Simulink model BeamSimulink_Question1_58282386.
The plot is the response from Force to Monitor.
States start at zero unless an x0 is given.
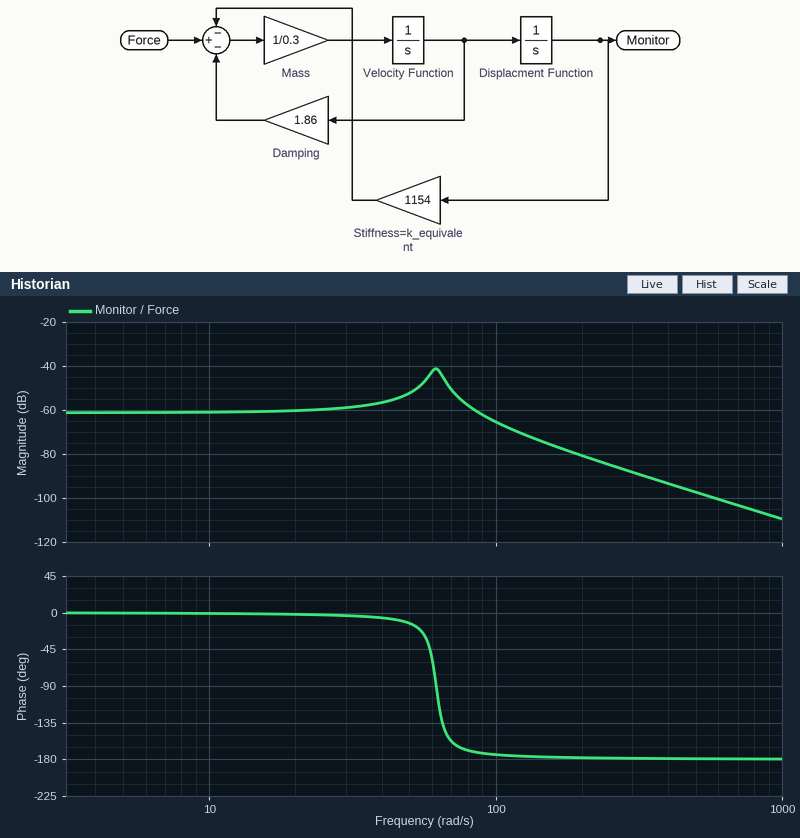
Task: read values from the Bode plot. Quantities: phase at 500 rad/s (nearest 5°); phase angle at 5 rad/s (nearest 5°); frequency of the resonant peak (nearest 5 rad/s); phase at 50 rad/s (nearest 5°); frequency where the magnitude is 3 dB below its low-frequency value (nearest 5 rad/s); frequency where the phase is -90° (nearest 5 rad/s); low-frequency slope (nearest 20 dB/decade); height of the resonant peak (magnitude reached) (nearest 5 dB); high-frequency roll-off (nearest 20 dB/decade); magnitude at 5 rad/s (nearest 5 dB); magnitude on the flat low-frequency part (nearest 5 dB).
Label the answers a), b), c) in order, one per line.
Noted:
a) -180°
b) 0°
c) 60 rad/s
d) -15°
e) 95 rad/s
f) 60 rad/s
g) 0 dB/decade
h) -40 dB
i) -40 dB/decade
j) -60 dB
k) -60 dB
